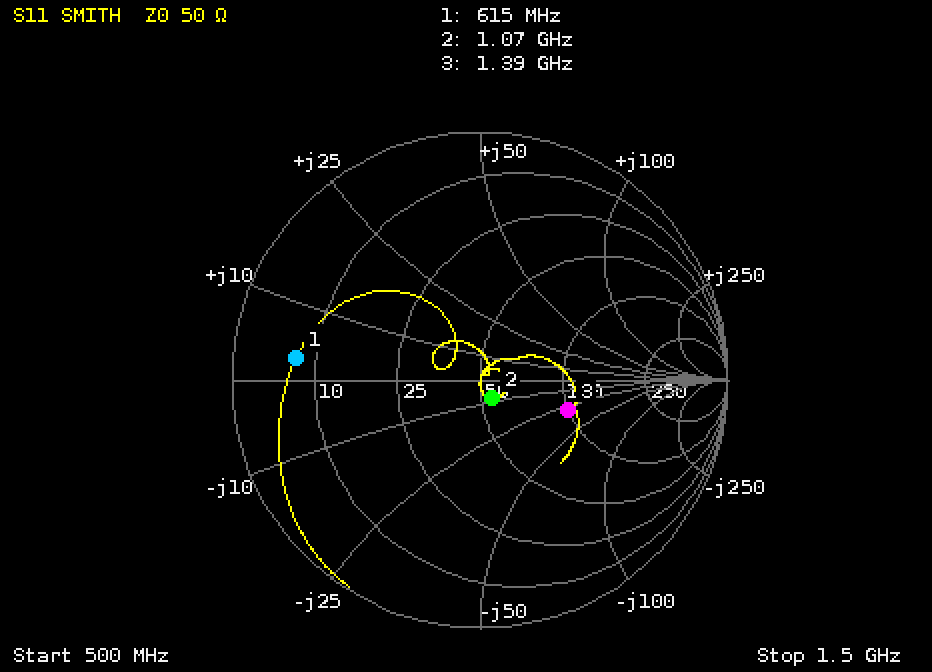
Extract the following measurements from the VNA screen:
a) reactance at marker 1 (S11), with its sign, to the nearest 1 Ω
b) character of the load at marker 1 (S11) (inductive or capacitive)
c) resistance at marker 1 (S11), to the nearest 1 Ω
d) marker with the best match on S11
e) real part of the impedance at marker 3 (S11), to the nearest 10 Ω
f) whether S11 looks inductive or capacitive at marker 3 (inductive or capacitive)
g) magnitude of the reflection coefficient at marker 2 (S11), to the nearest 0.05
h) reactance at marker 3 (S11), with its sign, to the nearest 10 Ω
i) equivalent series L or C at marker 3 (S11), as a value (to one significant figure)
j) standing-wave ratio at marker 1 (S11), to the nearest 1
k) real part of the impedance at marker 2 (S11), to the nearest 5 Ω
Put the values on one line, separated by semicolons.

+3 Ω; inductive; 7 Ω; marker 2; 100 Ω; capacitive; 0.10; -30 Ω; 4 pF; 7; 55 Ω
